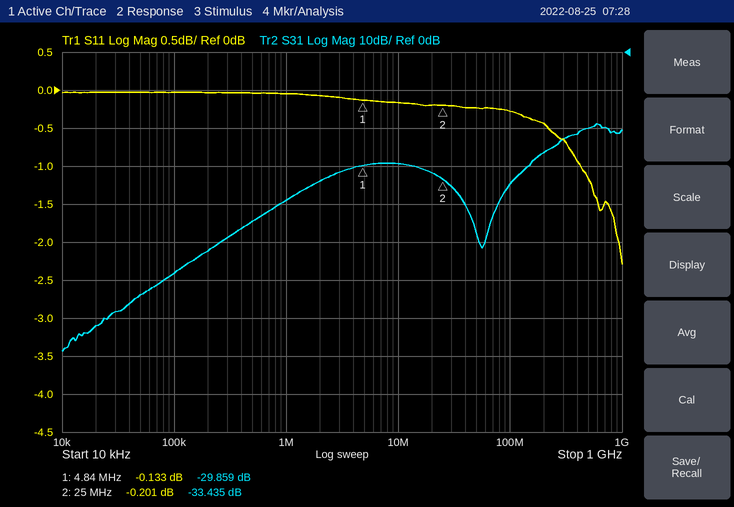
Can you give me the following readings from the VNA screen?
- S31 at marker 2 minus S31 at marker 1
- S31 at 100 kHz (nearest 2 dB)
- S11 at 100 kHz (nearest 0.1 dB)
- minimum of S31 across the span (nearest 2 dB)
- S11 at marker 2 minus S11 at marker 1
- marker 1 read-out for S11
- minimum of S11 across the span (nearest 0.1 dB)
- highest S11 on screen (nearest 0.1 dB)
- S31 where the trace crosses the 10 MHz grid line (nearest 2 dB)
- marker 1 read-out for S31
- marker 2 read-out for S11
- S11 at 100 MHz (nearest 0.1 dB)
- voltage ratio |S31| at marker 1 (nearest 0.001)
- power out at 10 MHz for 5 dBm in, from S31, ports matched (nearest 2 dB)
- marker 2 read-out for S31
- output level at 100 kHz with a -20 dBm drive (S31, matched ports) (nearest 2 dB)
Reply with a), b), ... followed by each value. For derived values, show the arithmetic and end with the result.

a) -33.435 − (-29.859) = -3.576 dB
b) -58 dB
c) 0.0 dB
d) -78 dB
e) -0.201 − (-0.133) = -0.068 dB
f) -0.133 dB
g) -2.3 dB
h) 0.0 dB
i) -30 dB
j) -29.859 dB
k) -0.201 dB
l) -0.3 dB
m) 10^(-29.859/20) ≈ 0.032
n) 5 dBm + (-30 dB) = -24 dBm
o) -33.435 dB
p) -20 dBm + (-58 dB) = -78 dBm
